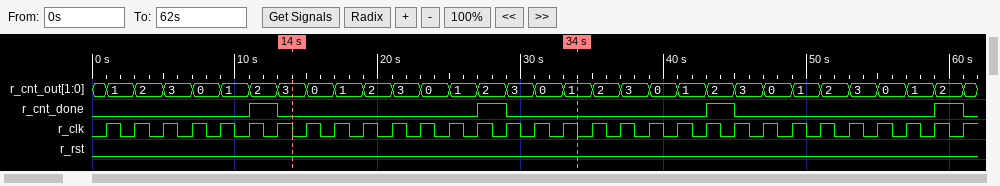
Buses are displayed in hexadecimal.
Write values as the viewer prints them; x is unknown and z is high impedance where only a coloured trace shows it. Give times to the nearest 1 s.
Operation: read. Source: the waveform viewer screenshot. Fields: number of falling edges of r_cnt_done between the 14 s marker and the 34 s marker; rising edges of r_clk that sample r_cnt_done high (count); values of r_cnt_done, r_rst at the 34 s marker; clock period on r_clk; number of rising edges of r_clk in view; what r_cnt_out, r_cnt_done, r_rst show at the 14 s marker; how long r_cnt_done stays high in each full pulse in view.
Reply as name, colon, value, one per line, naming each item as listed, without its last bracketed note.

number of falling edges of r_cnt_done between the 14 s marker and the 34 s marker: 1
rising edges of r_clk that sample r_cnt_done high: 4
values of r_cnt_done, r_rst at the 34 s marker: r_cnt_done=0, r_rst=0
clock period on r_clk: 2 s
number of rising edges of r_clk in view: 31
what r_cnt_out, r_cnt_done, r_rst show at the 14 s marker: r_cnt_out=3, r_cnt_done=0, r_rst=0
how long r_cnt_done stays high in each full pulse in view: 2 s, 2 s, 2 s, 2 s
